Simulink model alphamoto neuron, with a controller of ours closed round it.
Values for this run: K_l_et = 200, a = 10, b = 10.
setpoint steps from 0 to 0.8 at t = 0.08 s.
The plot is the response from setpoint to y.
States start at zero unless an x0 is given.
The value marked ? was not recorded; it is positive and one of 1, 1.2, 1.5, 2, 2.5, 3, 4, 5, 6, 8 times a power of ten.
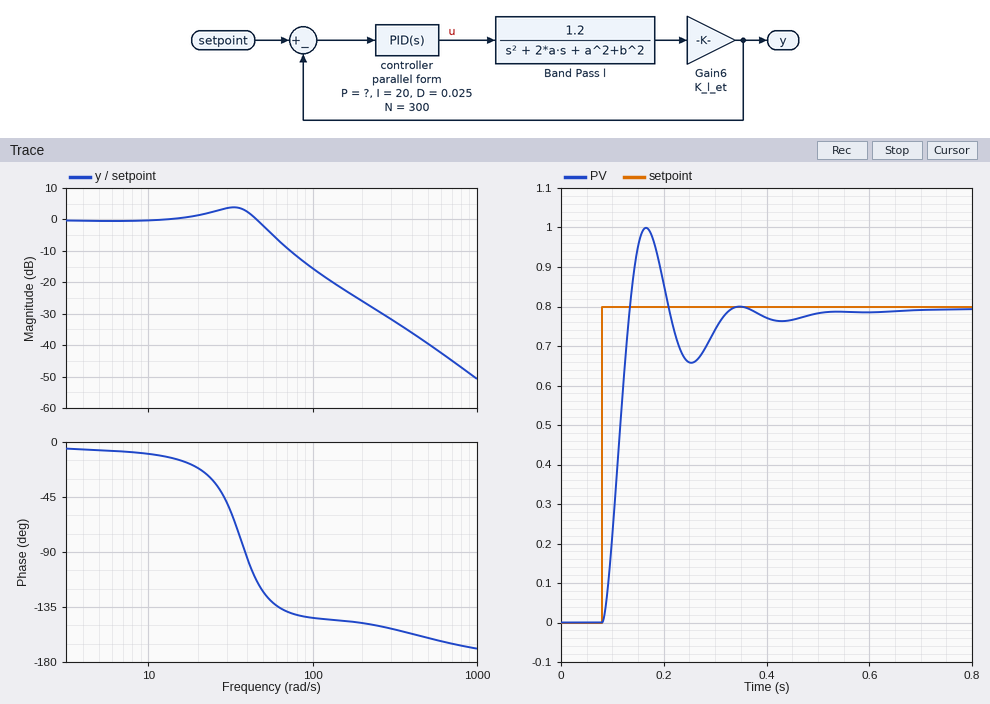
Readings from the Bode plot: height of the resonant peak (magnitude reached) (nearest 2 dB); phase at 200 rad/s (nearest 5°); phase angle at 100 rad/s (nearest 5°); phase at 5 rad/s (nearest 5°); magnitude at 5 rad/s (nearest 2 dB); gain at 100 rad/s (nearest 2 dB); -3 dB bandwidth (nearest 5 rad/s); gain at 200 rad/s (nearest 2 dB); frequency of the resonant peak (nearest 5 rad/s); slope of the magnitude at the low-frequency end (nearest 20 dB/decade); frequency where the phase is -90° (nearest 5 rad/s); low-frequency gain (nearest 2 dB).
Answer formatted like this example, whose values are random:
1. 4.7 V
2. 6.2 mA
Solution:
1. 4 dB
2. -150°
3. -145°
4. -5°
5. 0 dB
6. -16 dB
7. 55 rad/s
8. -26 dB
9. 35 rad/s
10. 0 dB/decade
11. 40 rad/s
12. 0 dB
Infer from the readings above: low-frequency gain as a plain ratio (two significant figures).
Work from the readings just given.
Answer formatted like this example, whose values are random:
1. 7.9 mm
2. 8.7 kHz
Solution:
1. 1.0
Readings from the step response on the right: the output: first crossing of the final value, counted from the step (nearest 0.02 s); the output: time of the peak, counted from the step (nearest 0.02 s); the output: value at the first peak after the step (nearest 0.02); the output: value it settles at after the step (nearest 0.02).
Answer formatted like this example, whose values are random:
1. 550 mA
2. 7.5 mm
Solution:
1. 0.06 s
2. 0.08 s
3. 1.00
4. 0.80
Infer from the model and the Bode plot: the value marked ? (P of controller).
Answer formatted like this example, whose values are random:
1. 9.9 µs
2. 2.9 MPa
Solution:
1. 5
